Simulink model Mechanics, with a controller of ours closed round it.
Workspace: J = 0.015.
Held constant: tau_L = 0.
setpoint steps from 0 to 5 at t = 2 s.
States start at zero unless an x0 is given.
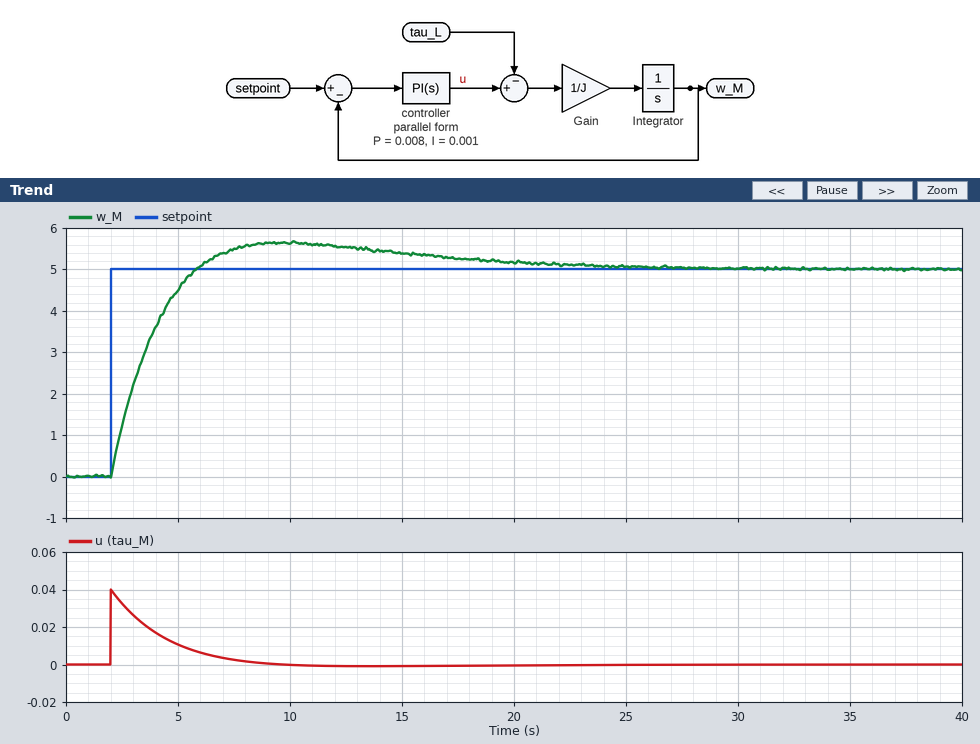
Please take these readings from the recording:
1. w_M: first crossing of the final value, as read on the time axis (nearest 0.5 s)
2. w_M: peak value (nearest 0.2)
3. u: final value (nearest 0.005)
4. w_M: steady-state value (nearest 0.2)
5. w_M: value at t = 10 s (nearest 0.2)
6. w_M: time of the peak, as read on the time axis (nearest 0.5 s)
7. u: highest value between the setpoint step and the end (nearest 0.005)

6.0 s
5.6
0.000
5.0
5.6
9.5 s
0.040
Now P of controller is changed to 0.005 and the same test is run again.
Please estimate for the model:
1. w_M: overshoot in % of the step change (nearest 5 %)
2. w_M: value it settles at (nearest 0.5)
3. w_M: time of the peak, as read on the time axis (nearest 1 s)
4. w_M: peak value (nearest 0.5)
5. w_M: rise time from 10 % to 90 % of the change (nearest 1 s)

25 %
5.0
11 s
6.0
3 s
